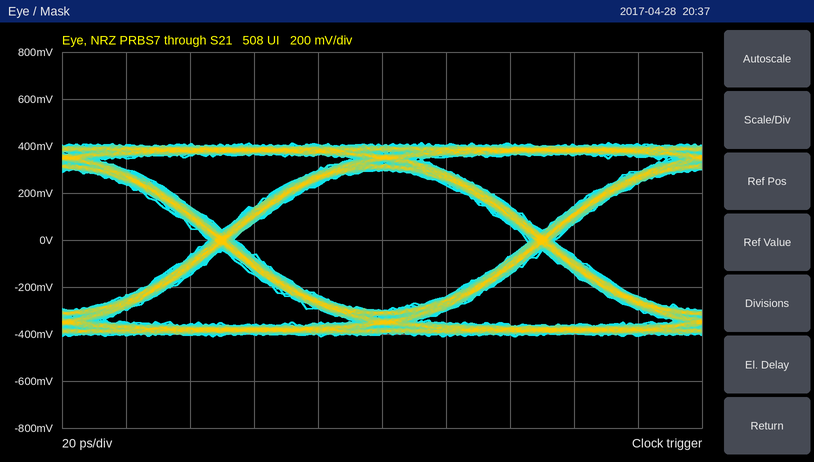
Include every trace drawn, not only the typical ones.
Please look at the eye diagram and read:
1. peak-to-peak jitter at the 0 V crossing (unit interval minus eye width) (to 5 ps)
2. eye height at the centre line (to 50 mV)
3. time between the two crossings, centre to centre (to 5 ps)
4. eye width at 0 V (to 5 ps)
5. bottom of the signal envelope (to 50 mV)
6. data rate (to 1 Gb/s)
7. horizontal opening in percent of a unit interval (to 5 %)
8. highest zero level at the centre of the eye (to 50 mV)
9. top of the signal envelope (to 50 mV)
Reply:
10 ps
600 mV
100 ps
90 ps
-400 mV
10 Gb/s
90 %
-300 mV
400 mV
